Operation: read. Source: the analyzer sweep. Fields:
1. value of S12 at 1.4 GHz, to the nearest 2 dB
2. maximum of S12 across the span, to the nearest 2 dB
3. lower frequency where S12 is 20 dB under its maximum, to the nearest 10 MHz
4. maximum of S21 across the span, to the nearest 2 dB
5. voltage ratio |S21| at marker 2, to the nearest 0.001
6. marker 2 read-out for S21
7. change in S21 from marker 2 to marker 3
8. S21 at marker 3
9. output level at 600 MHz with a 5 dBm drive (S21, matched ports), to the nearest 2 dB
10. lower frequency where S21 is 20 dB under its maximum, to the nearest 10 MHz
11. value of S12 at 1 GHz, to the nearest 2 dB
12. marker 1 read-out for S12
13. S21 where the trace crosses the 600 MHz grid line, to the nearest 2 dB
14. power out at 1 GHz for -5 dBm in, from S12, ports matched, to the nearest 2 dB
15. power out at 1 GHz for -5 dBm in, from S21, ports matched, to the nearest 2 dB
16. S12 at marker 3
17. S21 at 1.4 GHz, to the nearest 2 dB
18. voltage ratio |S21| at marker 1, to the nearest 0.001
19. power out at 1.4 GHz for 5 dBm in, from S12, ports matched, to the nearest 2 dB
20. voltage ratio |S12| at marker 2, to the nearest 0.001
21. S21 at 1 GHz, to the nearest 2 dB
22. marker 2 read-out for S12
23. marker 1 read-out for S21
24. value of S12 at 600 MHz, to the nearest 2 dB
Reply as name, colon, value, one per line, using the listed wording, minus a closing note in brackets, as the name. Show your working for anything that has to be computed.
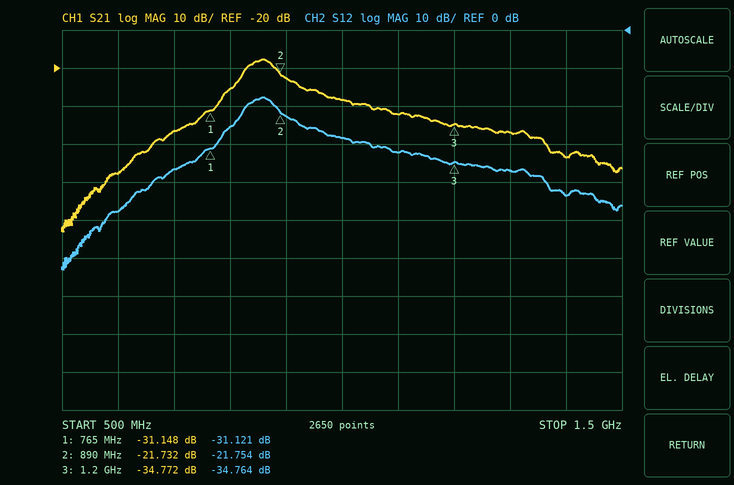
value of S12 at 1.4 GHz, to the nearest 2 dB: -44 dB
maximum of S12 across the span, to the nearest 2 dB: -18 dB
lower frequency where S12 is 20 dB under its maximum, to the nearest 10 MHz: 690 MHz
maximum of S21 across the span, to the nearest 2 dB: -18 dB
voltage ratio |S21| at marker 2, to the nearest 0.001: 10^(-21.732/20) ≈ 0.082
marker 2 read-out for S21: -21.732 dB
change in S21 from marker 2 to marker 3: -34.772 − (-21.732) = -13.040 dB
S21 at marker 3: -34.772 dB
output level at 600 MHz with a 5 dBm drive (S21, matched ports), to the nearest 2 dB: 5 dBm + (-48 dB) = -42 dBm
lower frequency where S21 is 20 dB under its maximum, to the nearest 10 MHz: 690 MHz
value of S12 at 1 GHz, to the nearest 2 dB: -28 dB
marker 1 read-out for S12: -31.121 dB
S21 where the trace crosses the 600 MHz grid line, to the nearest 2 dB: -48 dB
power out at 1 GHz for -5 dBm in, from S12, ports matched, to the nearest 2 dB: -5 dBm + (-28 dB) = -34 dBm
power out at 1 GHz for -5 dBm in, from S21, ports matched, to the nearest 2 dB: -5 dBm + (-28 dB) = -34 dBm
S12 at marker 3: -34.764 dB
S21 at 1.4 GHz, to the nearest 2 dB: -44 dB
voltage ratio |S21| at marker 1, to the nearest 0.001: 10^(-31.148/20) ≈ 0.028
power out at 1.4 GHz for 5 dBm in, from S12, ports matched, to the nearest 2 dB: 5 dBm + (-44 dB) = -38 dBm
voltage ratio |S12| at marker 2, to the nearest 0.001: 10^(-21.754/20) ≈ 0.082
S21 at 1 GHz, to the nearest 2 dB: -28 dB
marker 2 read-out for S12: -21.754 dB
marker 1 read-out for S21: -31.148 dB
value of S12 at 600 MHz, to the nearest 2 dB: -48 dB
